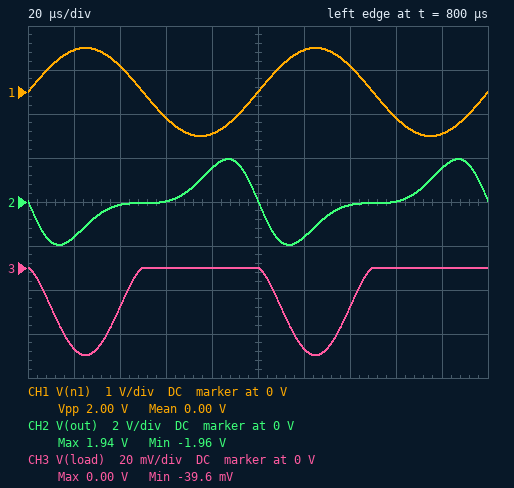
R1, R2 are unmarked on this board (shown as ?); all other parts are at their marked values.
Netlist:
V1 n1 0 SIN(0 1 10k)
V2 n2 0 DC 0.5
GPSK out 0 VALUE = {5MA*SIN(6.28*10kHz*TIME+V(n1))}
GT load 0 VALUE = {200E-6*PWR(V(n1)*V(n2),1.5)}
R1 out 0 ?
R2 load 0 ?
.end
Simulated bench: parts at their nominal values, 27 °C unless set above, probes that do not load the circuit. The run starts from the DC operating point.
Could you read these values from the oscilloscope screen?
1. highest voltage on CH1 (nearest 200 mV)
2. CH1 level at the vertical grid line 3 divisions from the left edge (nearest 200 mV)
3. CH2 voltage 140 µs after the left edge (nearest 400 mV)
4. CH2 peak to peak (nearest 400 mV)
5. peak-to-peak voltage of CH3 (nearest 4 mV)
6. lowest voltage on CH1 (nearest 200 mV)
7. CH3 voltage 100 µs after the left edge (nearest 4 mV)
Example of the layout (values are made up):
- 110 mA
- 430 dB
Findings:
- 1.0 V
- -600 mV
- 0 V
- 4.0 V
- 40 mV
- -1.0 V
- 0 V
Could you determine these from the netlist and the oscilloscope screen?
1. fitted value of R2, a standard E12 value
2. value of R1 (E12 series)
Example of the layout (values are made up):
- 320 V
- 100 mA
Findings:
- 560 Ω
- 390 Ω
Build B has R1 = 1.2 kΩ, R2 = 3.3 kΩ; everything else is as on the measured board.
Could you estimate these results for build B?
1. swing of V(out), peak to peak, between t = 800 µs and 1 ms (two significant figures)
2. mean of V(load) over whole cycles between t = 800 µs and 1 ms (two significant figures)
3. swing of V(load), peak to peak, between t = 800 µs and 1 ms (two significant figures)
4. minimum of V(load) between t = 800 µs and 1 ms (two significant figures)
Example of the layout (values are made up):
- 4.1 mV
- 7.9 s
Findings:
- 12 V
- -65 mV
- 230 mV
- -230 mV
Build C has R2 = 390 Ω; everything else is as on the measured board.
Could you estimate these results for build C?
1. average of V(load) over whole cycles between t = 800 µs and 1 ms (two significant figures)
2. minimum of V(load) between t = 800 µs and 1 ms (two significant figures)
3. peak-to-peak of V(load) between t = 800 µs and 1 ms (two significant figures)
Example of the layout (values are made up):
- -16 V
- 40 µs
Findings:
- -7.7 mV
- -28 mV
- 28 mV
